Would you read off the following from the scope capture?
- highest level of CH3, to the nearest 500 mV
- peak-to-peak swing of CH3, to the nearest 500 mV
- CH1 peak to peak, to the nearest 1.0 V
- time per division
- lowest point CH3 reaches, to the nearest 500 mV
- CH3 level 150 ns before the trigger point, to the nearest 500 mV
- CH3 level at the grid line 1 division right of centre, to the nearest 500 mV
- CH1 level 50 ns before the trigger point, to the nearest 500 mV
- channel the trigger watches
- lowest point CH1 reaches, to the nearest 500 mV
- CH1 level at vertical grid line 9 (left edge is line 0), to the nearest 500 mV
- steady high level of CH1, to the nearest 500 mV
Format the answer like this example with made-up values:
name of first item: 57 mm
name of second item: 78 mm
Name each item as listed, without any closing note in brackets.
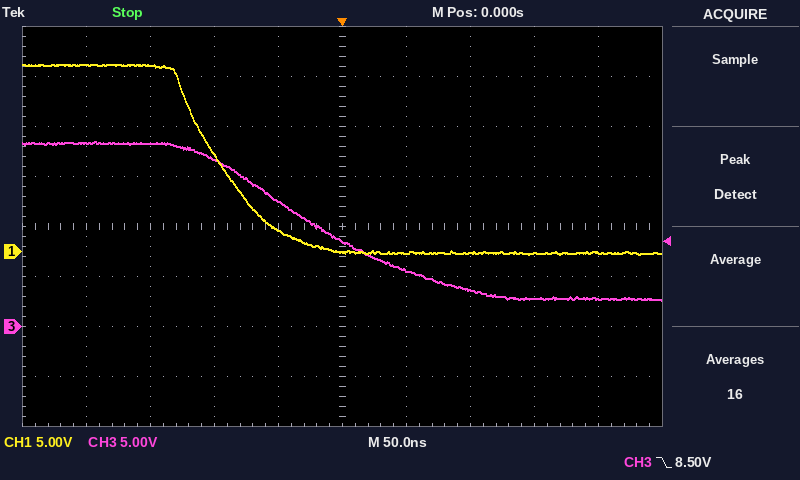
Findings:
highest level of CH3, to the nearest 500 mV: 18.5 V
peak-to-peak swing of CH3, to the nearest 500 mV: 16.0 V
CH1 peak to peak, to the nearest 1.0 V: 19.0 V
time per division: 50 ns
lowest point CH3 reaches, to the nearest 500 mV: 2.5 V
CH3 level 150 ns before the trigger point, to the nearest 500 mV: 18.5 V
CH3 level at the grid line 1 division right of centre, to the nearest 500 mV: 5.5 V
CH1 level 50 ns before the trigger point, to the nearest 500 mV: 2.0 V
channel the trigger watches: CH3
lowest point CH1 reaches, to the nearest 500 mV: -500 mV
CH1 level at vertical grid line 9 (left edge is line 0), to the nearest 500 mV: 0.0 V
steady high level of CH1, to the nearest 500 mV: 18.5 V
